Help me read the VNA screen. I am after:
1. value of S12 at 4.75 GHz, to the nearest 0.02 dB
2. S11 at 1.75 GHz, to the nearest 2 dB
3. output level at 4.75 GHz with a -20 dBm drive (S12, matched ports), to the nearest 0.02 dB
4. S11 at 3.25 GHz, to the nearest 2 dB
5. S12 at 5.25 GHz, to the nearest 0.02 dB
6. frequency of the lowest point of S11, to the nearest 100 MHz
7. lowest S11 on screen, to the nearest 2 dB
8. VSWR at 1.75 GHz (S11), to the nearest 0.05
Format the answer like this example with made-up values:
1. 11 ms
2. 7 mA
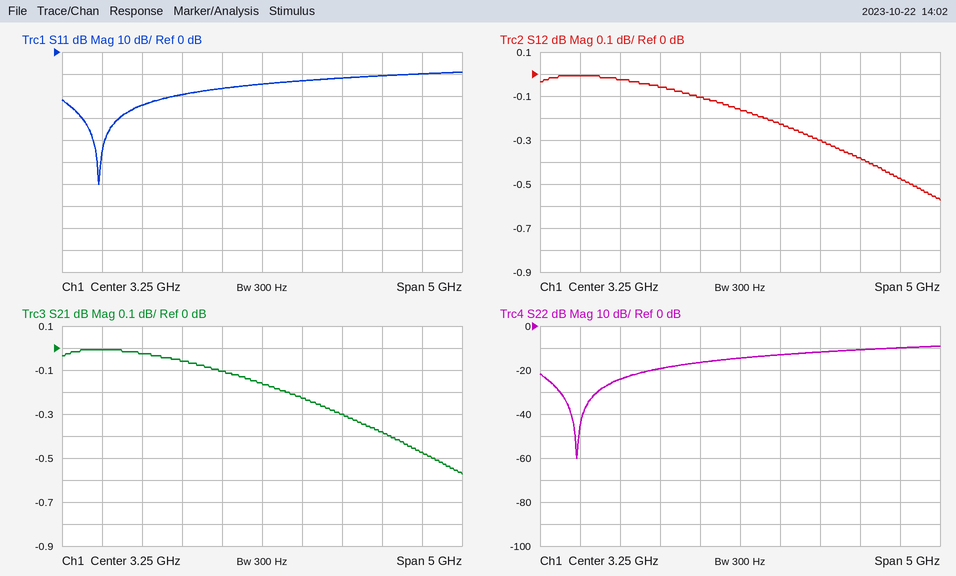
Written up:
1. -0.38 dB
2. -24 dB
3. -20.38 dBm
4. -14 dB
5. -0.48 dB
6. 1.2 GHz
7. -60 dB
8. 1.15
